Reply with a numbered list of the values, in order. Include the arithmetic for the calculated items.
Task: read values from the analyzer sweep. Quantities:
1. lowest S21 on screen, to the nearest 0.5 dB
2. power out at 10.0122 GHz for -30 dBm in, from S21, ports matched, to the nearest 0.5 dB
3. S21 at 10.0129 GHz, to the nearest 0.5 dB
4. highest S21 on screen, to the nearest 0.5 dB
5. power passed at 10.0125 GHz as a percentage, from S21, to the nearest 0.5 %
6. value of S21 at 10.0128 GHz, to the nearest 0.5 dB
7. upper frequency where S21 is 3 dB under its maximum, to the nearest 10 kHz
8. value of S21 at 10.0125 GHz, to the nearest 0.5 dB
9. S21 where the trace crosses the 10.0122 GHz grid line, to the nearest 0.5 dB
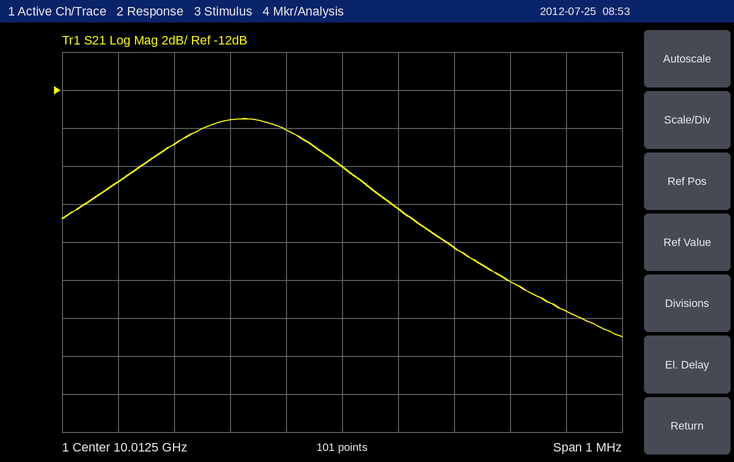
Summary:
1. -25.0 dB
2. -30 dBm + (-15.0 dB) = -45.0 dBm
3. -23.5 dB
4. -13.5 dB
5. 10^(-16/10) ≈ 2.5 %
6. -22.0 dB
7. 10.01252 GHz
8. -16.0 dB
9. -15.0 dB
